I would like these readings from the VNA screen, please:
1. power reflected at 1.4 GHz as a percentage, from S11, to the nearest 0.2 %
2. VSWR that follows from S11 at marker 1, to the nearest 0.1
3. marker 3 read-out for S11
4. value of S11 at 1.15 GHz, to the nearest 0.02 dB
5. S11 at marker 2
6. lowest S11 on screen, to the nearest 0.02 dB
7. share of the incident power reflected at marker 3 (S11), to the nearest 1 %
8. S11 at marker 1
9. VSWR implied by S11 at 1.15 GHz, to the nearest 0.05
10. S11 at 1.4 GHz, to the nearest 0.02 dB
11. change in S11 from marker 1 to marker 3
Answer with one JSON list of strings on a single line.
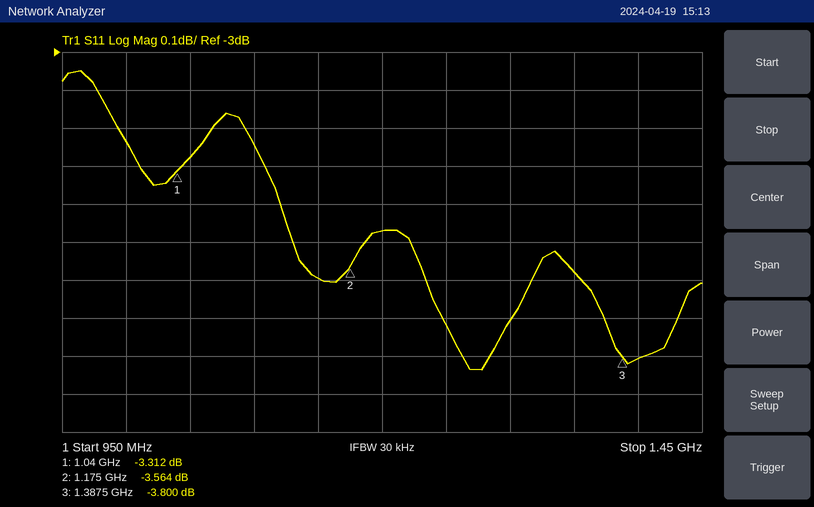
["41.6 %", "5.3", "-3.800 dB", "-3.60 dB", "-3.564 dB", "-3.84 dB", "42 %", "-3.312 dB", "4.90", "-3.80 dB", "-0.488 dB"]
